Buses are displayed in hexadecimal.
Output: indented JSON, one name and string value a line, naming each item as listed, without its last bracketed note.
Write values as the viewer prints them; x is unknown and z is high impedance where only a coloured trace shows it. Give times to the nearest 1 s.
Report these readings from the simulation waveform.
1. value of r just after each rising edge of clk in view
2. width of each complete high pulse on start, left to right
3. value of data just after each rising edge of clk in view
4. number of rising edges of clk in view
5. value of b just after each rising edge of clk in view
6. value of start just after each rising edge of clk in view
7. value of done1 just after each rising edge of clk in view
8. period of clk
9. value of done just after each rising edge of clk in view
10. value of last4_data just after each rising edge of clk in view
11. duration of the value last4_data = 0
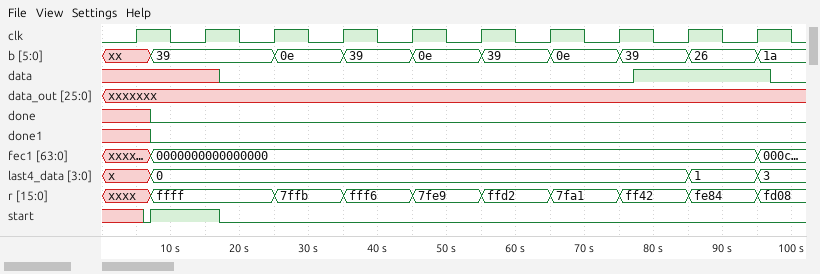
{
  "value of r just after each rising edge of clk in view": "xxxx, ffff, 7ffb, fff6, 7fe9, ffd2, 7fa1, ff42, fe84, fd08",
  "width of each complete high pulse on start, left to right": "10 s",
  "value of data just after each rising edge of clk in view": "x x 0 0 0 0 0 0 1 1",
  "number of rising edges of clk in view": "10",
  "value of b just after each rising edge of clk in view": "xx, 39, 0e, 39, 0e, 39, 0e, 39, 26, 1a",
  "value of start just after each rising edge of clk in view": "x 1 0 0 0 0 0 0 0 0",
  "value of done1 just after each rising edge of clk in view": "x 0 0 0 0 0 0 0 0 0",
  "period of clk": "10 s",
  "value of done just after each rising edge of clk in view": "x 0 0 0 0 0 0 0 0 0",
  "value of last4_data just after each rising edge of clk in view": "x, 0, 0, 0, 0, 0, 0, 0, 1, 3",
  "duration of the value last4_data = 0": "78 s"
}
